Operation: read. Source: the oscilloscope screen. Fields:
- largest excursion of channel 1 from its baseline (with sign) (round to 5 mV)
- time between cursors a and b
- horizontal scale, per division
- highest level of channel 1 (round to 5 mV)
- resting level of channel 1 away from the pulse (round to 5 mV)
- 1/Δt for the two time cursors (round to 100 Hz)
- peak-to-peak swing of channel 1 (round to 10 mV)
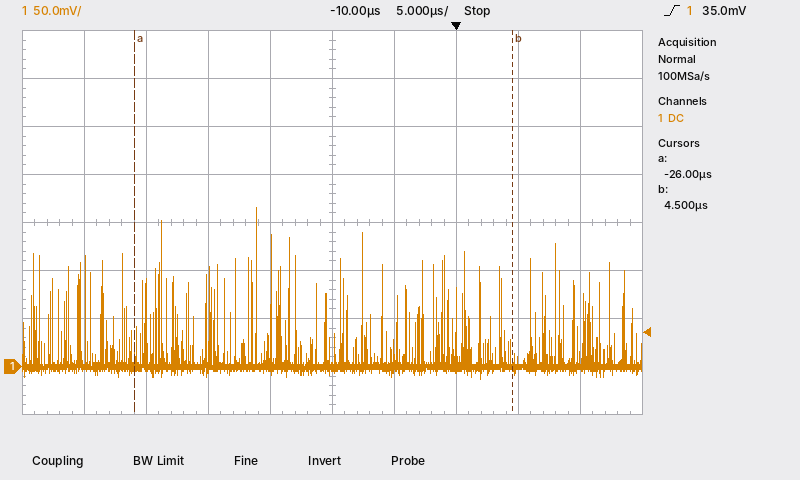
+165 mV
30.5 µs
5 µs
165 mV
0 mV
32.8 kHz
180 mV
